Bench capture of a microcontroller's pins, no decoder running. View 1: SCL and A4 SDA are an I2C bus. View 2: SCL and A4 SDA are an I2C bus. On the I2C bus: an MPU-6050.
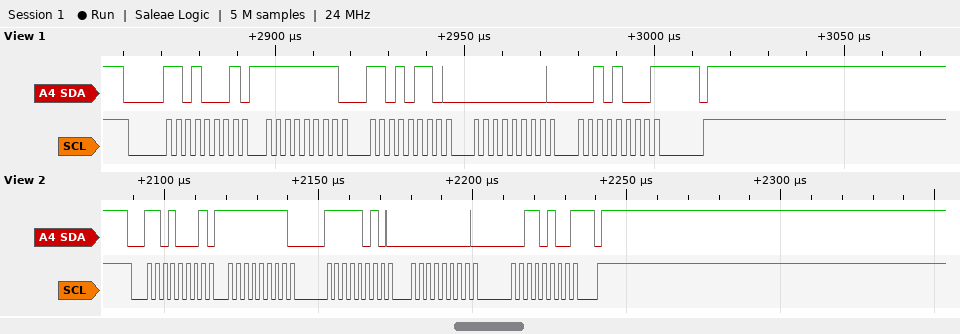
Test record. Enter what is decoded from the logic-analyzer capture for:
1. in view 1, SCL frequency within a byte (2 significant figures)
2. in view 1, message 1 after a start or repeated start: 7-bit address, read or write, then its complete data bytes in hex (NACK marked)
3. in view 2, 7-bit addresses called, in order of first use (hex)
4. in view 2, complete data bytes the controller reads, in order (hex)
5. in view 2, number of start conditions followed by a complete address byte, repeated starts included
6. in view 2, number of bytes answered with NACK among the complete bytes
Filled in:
400 kHz
0x68 read: FF D6 00 28 NACK
0x68
FF FA 00 34
1
1
